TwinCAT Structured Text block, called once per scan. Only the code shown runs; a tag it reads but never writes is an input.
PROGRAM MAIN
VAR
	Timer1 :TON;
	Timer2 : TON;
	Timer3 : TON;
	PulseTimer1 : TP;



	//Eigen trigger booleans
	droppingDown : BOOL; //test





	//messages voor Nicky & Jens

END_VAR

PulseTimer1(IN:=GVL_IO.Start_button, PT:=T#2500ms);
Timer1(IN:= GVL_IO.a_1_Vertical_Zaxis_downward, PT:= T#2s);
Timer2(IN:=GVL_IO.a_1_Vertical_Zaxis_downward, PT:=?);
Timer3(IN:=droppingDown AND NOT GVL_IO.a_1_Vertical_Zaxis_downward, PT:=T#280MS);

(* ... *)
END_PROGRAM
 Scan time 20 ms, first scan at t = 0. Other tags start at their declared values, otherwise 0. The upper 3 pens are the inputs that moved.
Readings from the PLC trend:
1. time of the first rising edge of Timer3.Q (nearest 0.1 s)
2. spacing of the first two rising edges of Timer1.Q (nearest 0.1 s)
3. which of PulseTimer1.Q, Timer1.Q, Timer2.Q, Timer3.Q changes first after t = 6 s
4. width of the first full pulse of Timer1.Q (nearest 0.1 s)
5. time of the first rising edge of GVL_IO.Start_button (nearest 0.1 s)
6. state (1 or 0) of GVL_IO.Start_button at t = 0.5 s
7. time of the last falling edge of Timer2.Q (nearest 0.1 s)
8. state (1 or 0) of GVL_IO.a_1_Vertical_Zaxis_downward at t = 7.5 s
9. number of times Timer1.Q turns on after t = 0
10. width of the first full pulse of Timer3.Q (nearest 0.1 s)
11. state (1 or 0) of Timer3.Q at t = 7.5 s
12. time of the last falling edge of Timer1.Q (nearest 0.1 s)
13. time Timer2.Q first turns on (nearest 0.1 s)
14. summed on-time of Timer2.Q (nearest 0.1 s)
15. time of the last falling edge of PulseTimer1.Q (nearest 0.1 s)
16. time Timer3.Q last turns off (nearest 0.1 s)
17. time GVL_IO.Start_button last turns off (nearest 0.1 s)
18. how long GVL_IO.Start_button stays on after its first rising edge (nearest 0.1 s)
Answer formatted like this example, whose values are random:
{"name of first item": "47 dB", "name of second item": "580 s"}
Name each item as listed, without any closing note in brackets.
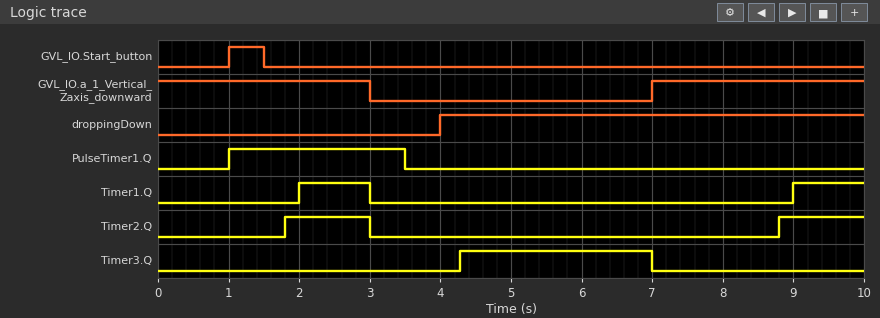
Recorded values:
{"time of the first rising edge of Timer3.Q": "4.3 s", "spacing of the first two rising edges of Timer1.Q": "7.0 s", "which of PulseTimer1.Q, Timer1.Q, Timer2.Q, Timer3.Q changes first after t = 6 s": "Timer3.Q", "width of the first full pulse of Timer1.Q": "1.0 s", "time of the first rising edge of GVL_IO.Start_button": "1.0 s", "state (1 or 0) of GVL_IO.Start_button at t = 0.5 s": "0", "time of the last falling edge of Timer2.Q": "3.0 s", "state (1 or 0) of GVL_IO.a_1_Vertical_Zaxis_downward at t = 7.5 s": "1", "number of times Timer1.Q turns on after t = 0": "2", "width of the first full pulse of Timer3.Q": "2.7 s", "state (1 or 0) of Timer3.Q at t = 7.5 s": "0", "time of the last falling edge of Timer1.Q": "3.0 s", "time Timer2.Q first turns on": "1.8 s", "summed on-time of Timer2.Q": "2.4 s", "time of the last falling edge of PulseTimer1.Q": "3.5 s", "time Timer3.Q last turns off": "7.0 s", "time GVL_IO.Start_button last turns off": "1.5 s", "how long GVL_IO.Start_button stays on after its first rising edge": "0.5 s"}
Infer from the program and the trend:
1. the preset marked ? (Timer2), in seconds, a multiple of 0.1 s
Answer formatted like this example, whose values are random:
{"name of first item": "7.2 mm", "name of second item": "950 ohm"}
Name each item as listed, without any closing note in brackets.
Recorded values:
{"the preset marked ? (Timer2), in seconds, a multiple of 0.1 s": "1.8 s"}
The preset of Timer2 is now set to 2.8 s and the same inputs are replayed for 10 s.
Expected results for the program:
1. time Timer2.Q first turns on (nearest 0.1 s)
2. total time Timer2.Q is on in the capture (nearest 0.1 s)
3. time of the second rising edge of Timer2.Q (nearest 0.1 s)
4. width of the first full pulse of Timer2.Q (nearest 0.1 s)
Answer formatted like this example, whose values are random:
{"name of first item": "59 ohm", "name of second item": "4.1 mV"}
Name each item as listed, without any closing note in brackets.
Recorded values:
{"time Timer2.Q first turns on": "2.8 s", "total time Timer2.Q is on in the capture": "0.4 s", "time of the second rising edge of Timer2.Q": "9.8 s", "width of the first full pulse of Timer2.Q": "0.2 s"}
